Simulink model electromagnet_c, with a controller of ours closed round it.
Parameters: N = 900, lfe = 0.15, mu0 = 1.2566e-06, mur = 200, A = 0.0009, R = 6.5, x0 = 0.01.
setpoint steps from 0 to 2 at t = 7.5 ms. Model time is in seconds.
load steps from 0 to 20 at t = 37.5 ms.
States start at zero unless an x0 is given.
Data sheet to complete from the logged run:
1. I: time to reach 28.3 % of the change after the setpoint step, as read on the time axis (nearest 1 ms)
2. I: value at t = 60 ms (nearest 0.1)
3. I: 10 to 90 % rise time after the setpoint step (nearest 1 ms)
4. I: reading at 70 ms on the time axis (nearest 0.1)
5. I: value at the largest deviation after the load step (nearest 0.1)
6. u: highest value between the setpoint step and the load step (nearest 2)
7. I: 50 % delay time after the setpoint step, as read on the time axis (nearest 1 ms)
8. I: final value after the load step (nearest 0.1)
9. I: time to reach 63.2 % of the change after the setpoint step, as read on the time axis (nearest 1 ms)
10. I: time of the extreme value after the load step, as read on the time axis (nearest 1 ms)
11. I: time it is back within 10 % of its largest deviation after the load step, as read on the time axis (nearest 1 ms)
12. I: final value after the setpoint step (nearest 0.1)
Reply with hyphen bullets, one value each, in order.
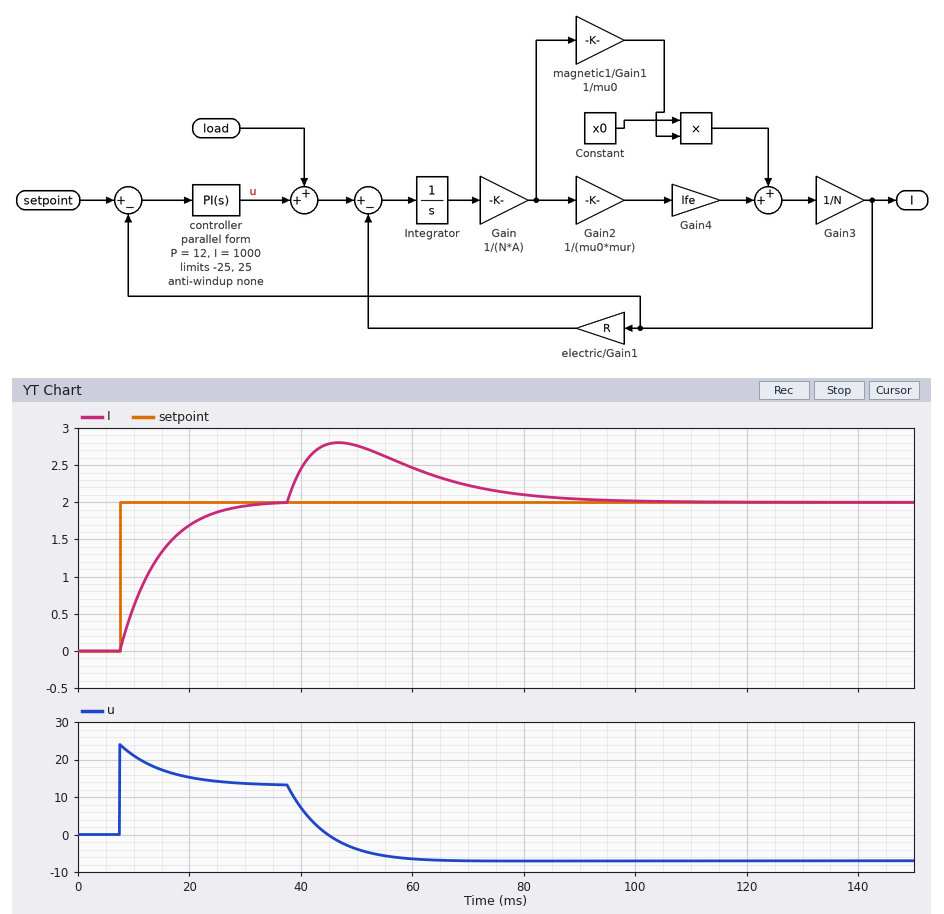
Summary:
- 10 ms
- 2.5
- 14 ms
- 2.2
- 2.8
- 24
- 12 ms
- 2.0
- 14 ms
- 47 ms
- 83 ms
- 2.0
